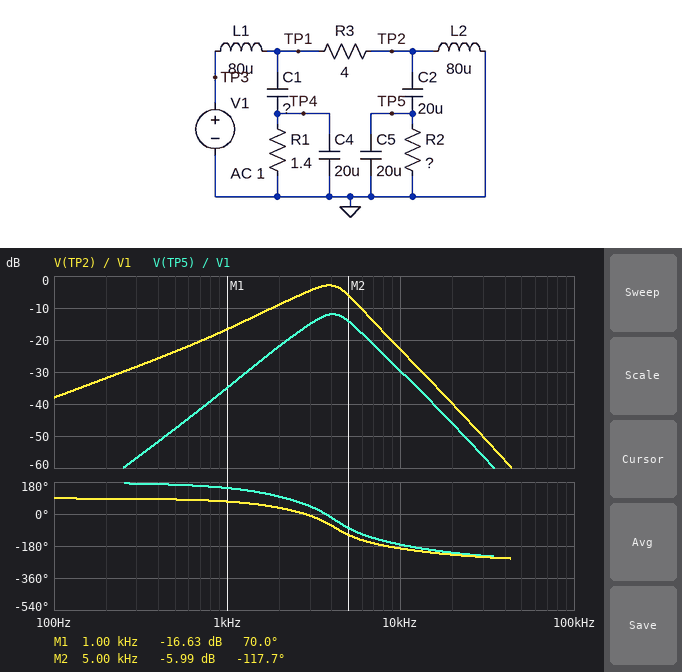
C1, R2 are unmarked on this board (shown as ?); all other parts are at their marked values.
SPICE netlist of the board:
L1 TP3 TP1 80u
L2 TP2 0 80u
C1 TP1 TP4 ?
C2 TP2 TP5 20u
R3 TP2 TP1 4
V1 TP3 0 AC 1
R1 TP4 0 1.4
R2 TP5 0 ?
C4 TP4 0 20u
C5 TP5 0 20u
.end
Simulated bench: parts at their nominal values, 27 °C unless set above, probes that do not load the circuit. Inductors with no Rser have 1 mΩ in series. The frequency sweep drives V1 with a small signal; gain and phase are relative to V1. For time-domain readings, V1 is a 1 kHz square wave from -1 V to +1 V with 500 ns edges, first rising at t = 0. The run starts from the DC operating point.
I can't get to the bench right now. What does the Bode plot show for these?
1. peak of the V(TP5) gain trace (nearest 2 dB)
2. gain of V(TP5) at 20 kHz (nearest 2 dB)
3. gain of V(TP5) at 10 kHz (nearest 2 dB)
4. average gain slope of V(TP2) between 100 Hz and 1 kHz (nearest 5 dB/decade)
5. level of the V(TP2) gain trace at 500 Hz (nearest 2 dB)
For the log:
-12 dB
-46 dB
-30 dB
20 dB/decade
-24 dB
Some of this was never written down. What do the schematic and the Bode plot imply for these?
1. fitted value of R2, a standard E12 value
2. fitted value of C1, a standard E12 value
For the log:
1 Ω
56 µF
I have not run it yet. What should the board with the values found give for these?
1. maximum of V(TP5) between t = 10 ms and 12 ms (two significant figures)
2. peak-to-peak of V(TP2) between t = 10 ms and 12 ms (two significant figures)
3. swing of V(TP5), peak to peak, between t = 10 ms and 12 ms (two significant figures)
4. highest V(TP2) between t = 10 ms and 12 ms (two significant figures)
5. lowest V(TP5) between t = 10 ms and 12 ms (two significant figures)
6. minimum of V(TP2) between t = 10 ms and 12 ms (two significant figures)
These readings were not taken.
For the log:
130 mV
1.2 V
270 mV
580 mV
-130 mV
-580 mV
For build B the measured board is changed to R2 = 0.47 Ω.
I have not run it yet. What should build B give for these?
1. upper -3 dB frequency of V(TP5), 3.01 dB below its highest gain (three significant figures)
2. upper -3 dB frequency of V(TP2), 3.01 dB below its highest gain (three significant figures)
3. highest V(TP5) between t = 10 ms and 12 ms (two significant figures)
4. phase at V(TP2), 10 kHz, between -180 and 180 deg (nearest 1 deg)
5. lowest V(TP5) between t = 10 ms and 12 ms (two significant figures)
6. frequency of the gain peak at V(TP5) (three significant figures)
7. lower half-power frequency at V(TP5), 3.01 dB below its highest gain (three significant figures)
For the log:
4.82 kHz
4.57 kHz
83 mV
164 deg
-83 mV
3.94 kHz
3.19 kHz
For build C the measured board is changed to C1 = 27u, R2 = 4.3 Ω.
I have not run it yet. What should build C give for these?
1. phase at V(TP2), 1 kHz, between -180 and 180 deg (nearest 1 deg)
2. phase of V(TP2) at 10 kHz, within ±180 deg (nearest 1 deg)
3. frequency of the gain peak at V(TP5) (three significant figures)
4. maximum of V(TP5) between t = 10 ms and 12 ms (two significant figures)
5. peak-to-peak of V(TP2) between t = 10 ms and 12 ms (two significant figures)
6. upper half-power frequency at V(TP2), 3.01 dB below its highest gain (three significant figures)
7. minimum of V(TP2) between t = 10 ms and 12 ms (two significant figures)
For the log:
73 deg
156 deg
4.98 kHz
330 mV
1.6 V
5.81 kHz
-790 mV
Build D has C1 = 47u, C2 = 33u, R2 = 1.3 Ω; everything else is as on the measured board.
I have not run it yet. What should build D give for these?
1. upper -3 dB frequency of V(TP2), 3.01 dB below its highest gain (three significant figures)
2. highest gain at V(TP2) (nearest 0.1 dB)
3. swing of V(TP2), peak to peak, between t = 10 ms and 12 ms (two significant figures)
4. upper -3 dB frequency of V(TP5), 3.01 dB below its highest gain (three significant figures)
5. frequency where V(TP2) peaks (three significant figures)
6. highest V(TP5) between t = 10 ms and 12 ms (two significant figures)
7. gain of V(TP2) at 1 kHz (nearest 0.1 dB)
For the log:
4.73 kHz
-3.6 dB
1.1 V
4.88 kHz
3.54 kHz
200 mV
-16.5 dB
